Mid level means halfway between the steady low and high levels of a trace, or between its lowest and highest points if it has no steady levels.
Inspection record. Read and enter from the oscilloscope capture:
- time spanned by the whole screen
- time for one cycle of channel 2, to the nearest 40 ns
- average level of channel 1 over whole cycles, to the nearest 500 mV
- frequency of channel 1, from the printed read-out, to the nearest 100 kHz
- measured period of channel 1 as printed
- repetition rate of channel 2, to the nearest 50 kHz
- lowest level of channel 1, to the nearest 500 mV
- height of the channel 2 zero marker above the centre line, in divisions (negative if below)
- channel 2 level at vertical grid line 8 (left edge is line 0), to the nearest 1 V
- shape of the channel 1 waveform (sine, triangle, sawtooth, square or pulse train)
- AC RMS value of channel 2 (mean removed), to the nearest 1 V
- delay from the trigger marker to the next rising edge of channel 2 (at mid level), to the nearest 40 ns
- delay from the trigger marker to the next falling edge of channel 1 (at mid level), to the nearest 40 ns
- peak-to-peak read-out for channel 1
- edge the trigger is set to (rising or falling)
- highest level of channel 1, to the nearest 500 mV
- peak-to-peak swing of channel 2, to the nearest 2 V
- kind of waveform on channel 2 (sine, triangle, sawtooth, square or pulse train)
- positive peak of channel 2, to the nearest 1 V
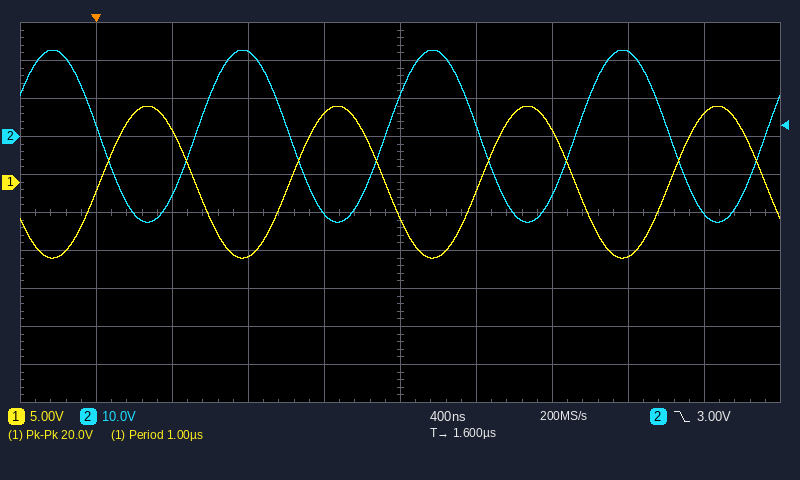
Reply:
4 µs
1.00 µs
0.0 V
1.0 MHz
1.00 µs
1.00 MHz
-10.0 V
+2.0 div
22 V
sine
16 V
520 ns
520 ns
20.0 V
falling
10.0 V
46 V
sine
23 V
